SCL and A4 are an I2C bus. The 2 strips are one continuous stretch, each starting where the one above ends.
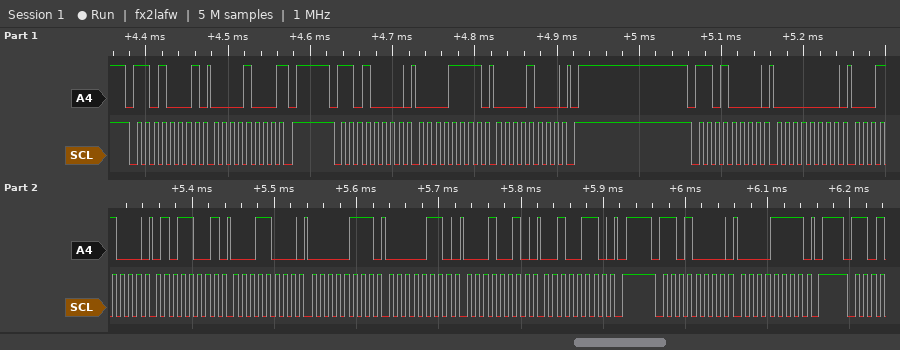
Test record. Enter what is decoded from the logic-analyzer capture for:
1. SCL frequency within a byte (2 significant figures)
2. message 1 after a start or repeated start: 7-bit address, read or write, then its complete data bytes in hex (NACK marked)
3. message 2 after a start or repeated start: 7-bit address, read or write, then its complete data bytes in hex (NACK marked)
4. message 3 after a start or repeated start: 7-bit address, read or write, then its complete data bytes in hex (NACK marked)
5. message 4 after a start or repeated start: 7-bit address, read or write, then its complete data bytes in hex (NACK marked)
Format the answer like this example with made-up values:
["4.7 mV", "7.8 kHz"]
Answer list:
["100 kHz", "0x68 read: 08 NACK", "0x68 write: 0F 08", "0x68 write: 00 18 59 18 07 06 12 26", "0x68 write: 0F"]
